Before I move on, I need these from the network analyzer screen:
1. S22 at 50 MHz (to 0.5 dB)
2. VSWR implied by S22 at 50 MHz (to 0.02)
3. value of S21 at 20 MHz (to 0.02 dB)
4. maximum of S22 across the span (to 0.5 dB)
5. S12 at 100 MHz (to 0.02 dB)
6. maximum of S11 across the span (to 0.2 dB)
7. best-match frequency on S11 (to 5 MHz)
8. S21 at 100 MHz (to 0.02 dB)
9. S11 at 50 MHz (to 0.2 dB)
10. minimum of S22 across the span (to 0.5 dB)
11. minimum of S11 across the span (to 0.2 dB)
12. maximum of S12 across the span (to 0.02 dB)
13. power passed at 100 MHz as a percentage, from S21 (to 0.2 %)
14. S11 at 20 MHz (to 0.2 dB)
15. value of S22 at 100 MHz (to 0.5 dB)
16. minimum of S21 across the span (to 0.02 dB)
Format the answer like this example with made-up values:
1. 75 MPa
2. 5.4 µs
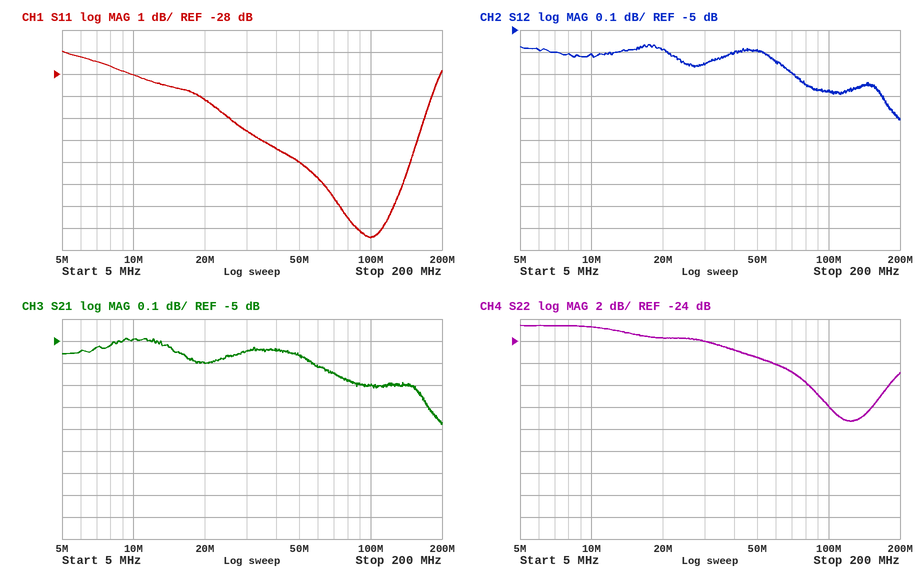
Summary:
1. -25.5 dB
2. 1.12
3. -5.10 dB
4. -22.5 dB
5. -5.28 dB
6. -27.0 dB
7. 100 MHz
8. -5.20 dB
9. -32.0 dB
10. -31.5 dB
11. -35.4 dB
12. -5.06 dB
13. 30.2 %
14. -29.2 dB
15. -30.0 dB
16. -5.38 dB
